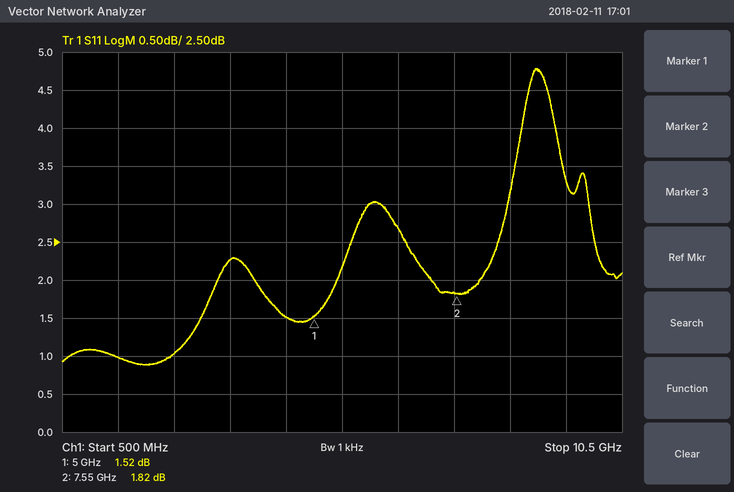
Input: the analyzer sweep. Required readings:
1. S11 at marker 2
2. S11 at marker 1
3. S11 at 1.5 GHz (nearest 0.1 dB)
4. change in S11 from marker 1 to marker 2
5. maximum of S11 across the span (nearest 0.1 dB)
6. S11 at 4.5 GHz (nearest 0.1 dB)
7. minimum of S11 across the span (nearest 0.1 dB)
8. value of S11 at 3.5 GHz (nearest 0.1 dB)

1.82 dB
1.52 dB
1.0 dB
0.30 dB
4.8 dB
1.5 dB
0.9 dB
2.3 dB
